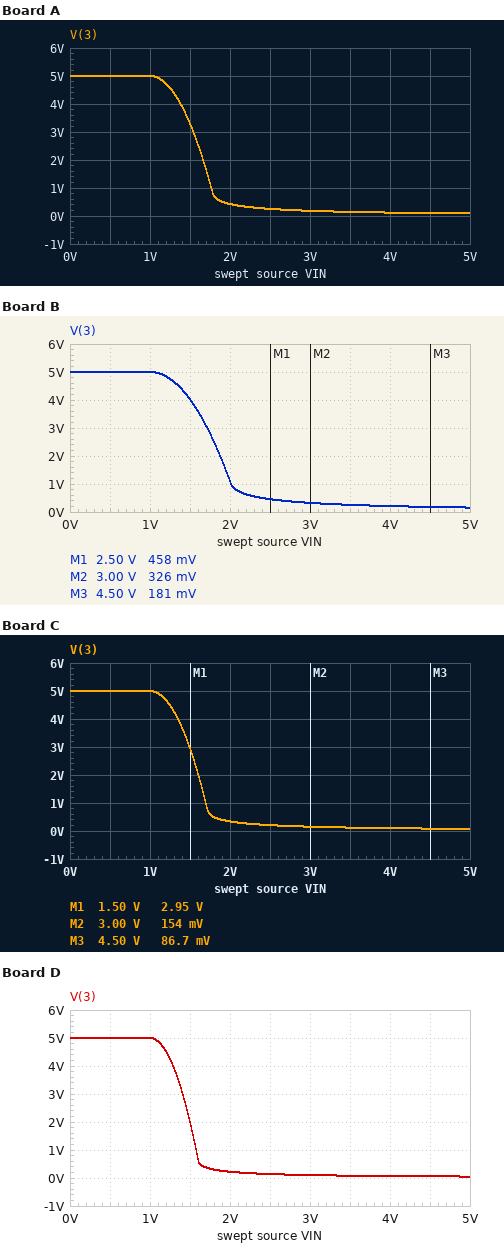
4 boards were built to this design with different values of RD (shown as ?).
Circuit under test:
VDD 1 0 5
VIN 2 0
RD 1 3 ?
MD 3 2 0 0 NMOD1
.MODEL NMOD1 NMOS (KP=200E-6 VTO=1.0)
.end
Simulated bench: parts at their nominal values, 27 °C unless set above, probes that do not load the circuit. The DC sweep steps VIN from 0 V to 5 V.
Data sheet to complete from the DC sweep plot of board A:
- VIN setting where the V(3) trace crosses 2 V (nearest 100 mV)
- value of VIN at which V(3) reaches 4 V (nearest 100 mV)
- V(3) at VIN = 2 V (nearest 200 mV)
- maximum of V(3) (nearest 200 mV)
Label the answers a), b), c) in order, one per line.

a) 1.7 V
b) 1.4 V
c) 400 mV
d) 5.0 V
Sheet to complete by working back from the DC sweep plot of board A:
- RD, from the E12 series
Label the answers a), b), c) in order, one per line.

a) 68 kΩ
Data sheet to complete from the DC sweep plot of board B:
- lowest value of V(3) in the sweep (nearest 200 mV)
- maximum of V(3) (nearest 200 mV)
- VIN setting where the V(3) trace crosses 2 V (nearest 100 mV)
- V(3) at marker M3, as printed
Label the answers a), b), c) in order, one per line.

a) 200 mV
b) 5.0 V
c) 1.9 V
d) 181 mV
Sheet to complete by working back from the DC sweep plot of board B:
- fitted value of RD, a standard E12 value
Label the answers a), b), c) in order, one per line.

a) 39 kΩ
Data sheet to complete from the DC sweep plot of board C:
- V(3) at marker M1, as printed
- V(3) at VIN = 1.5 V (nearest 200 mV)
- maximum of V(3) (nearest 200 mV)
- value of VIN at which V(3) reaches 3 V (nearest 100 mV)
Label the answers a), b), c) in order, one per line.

a) 2.95 V
b) 3.0 V
c) 5.0 V
d) 1.5 V
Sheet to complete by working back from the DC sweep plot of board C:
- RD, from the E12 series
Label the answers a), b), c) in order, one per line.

a) 82 kΩ
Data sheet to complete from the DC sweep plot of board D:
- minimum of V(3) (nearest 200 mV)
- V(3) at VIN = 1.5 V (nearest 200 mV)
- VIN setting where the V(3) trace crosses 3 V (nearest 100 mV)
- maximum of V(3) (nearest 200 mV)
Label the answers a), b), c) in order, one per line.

a) 0 V
b) 2.0 V
c) 1.4 V
d) 5.0 V
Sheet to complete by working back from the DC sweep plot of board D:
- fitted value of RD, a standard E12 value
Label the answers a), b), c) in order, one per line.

a) 120 kΩ
